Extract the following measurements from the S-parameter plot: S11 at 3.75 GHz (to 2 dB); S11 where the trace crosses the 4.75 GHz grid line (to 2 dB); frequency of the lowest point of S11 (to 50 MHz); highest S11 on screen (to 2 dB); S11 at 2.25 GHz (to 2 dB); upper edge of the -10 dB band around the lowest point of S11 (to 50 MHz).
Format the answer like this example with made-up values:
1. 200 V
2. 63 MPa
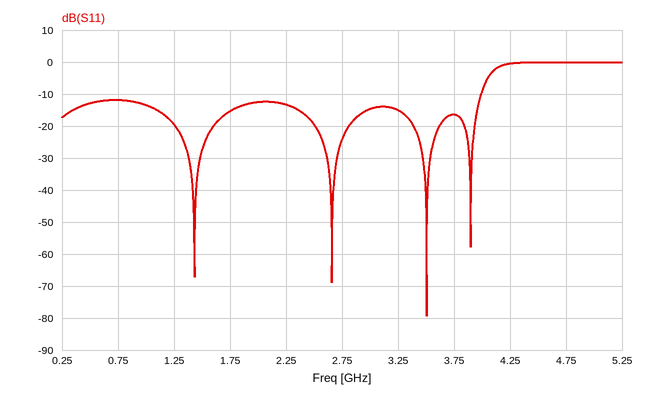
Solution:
1. -16 dB
2. 0 dB
3. 3.50 GHz
4. 0 dB
5. -14 dB
6. 4.00 GHz
